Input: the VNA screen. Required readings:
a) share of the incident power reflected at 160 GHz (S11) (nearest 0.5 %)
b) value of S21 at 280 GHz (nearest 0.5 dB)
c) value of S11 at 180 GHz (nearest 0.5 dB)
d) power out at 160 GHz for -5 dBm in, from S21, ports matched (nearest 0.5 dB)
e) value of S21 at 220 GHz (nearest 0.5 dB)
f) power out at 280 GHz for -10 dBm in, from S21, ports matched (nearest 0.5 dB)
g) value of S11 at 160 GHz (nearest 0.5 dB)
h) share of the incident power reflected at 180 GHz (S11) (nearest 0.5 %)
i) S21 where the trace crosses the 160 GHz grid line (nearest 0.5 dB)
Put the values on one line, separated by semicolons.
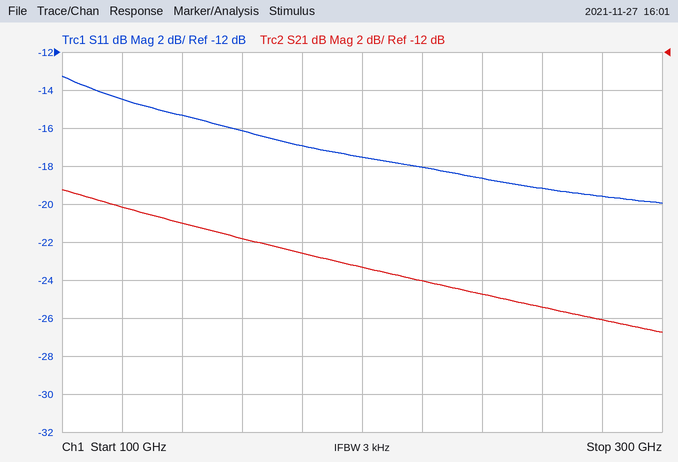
2.5 %; -26.0 dB; -17.0 dB; -27.0 dBm; -24.0 dB; -36.0 dBm; -16.0 dB; 2.0 %; -22.0 dB
